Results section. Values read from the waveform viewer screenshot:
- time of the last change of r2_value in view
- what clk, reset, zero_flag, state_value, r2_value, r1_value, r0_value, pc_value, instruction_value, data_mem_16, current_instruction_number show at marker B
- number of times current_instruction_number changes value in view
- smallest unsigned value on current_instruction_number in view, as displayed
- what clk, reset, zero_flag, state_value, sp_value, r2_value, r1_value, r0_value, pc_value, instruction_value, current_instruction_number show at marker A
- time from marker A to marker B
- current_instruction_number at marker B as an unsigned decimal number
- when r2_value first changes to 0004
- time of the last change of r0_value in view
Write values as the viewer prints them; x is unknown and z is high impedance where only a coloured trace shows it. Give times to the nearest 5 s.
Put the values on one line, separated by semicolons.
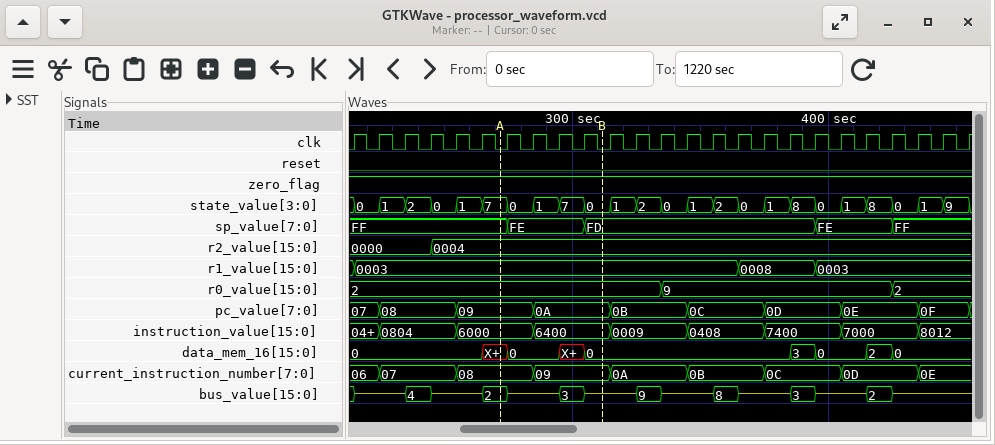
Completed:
245 s; clk=0, reset=0, zero_flag=1, state_value=0, r2_value=0004, r1_value=0003, r0_value=2, pc_value=0A, instruction_value=6400, data_mem_16=0, current_instruction_number=09; 8; 06; clk=0, reset=0, zero_flag=1, state_value=7, sp_value=FF, r2_value=0004, r1_value=0003, r0_value=2, pc_value=09, instruction_value=6000, current_instruction_number=08; 40 s; 9; 245 s; 425 s
